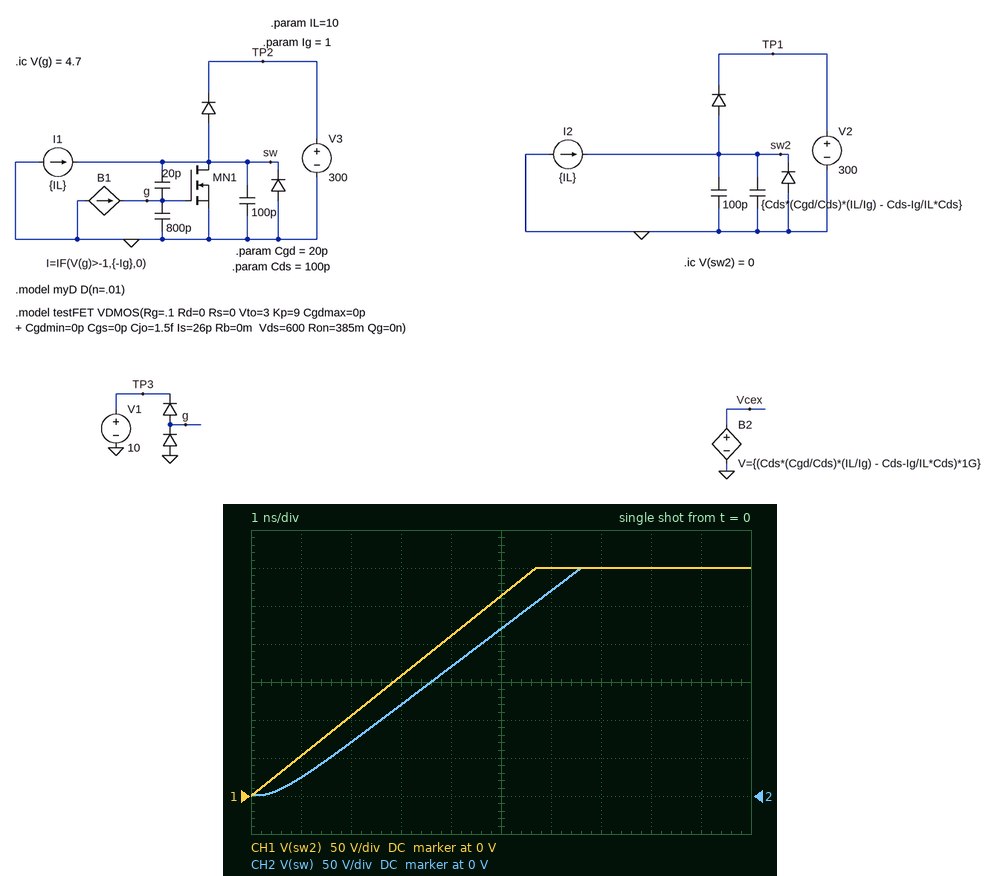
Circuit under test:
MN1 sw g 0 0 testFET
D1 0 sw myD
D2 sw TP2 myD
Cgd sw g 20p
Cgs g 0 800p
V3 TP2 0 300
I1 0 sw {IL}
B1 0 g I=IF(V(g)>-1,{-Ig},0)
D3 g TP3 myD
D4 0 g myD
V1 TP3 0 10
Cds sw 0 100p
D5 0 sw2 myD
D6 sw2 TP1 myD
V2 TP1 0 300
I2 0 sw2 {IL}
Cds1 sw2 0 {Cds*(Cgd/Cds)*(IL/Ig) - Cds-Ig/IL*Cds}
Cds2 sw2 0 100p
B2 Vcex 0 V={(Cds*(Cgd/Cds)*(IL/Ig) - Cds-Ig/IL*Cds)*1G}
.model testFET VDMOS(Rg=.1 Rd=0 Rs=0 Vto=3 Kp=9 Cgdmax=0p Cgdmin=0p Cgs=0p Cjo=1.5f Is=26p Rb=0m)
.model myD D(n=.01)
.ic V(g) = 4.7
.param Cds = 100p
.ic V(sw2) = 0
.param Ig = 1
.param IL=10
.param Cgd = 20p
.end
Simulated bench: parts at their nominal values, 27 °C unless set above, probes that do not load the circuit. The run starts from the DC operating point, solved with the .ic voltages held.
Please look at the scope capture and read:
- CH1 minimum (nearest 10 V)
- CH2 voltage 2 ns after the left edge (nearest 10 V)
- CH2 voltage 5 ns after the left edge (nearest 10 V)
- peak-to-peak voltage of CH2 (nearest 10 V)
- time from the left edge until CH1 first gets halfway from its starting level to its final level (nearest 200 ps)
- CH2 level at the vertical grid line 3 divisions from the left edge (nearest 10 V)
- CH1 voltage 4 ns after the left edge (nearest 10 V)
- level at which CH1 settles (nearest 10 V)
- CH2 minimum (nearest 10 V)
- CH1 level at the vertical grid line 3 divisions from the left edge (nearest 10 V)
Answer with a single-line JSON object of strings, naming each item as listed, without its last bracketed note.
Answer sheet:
{"CH1 minimum": "0 V", "CH2 voltage 2 ns after the left edge": "70 V", "CH2 voltage 5 ns after the left edge": "220 V", "peak-to-peak voltage of CH2": "300 V", "time from the left edge until CH1 first gets halfway from its starting level to its final level": "2.8 ns", "CH2 level at the vertical grid line 3 divisions from the left edge": "120 V", "CH1 voltage 4 ns after the left edge": "210 V", "level at which CH1 settles": "300 V", "CH2 minimum": "0 V", "CH1 level at the vertical grid line 3 divisions from the left edge": "160 V"}
